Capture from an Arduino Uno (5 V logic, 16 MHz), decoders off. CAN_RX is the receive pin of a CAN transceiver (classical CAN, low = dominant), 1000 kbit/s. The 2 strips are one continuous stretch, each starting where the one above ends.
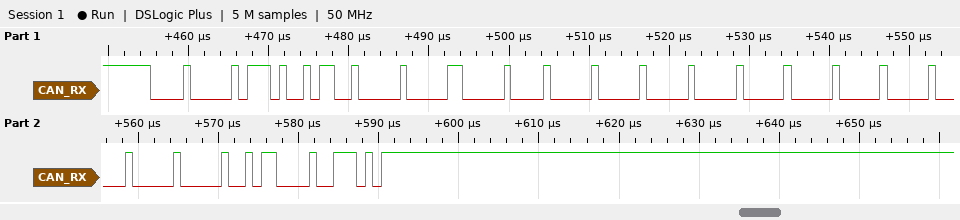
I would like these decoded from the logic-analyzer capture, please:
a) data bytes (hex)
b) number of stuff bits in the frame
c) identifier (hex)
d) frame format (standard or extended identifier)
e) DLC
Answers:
02 00 00 00 00 00 00 00
15
0x02052C80
extended
8
